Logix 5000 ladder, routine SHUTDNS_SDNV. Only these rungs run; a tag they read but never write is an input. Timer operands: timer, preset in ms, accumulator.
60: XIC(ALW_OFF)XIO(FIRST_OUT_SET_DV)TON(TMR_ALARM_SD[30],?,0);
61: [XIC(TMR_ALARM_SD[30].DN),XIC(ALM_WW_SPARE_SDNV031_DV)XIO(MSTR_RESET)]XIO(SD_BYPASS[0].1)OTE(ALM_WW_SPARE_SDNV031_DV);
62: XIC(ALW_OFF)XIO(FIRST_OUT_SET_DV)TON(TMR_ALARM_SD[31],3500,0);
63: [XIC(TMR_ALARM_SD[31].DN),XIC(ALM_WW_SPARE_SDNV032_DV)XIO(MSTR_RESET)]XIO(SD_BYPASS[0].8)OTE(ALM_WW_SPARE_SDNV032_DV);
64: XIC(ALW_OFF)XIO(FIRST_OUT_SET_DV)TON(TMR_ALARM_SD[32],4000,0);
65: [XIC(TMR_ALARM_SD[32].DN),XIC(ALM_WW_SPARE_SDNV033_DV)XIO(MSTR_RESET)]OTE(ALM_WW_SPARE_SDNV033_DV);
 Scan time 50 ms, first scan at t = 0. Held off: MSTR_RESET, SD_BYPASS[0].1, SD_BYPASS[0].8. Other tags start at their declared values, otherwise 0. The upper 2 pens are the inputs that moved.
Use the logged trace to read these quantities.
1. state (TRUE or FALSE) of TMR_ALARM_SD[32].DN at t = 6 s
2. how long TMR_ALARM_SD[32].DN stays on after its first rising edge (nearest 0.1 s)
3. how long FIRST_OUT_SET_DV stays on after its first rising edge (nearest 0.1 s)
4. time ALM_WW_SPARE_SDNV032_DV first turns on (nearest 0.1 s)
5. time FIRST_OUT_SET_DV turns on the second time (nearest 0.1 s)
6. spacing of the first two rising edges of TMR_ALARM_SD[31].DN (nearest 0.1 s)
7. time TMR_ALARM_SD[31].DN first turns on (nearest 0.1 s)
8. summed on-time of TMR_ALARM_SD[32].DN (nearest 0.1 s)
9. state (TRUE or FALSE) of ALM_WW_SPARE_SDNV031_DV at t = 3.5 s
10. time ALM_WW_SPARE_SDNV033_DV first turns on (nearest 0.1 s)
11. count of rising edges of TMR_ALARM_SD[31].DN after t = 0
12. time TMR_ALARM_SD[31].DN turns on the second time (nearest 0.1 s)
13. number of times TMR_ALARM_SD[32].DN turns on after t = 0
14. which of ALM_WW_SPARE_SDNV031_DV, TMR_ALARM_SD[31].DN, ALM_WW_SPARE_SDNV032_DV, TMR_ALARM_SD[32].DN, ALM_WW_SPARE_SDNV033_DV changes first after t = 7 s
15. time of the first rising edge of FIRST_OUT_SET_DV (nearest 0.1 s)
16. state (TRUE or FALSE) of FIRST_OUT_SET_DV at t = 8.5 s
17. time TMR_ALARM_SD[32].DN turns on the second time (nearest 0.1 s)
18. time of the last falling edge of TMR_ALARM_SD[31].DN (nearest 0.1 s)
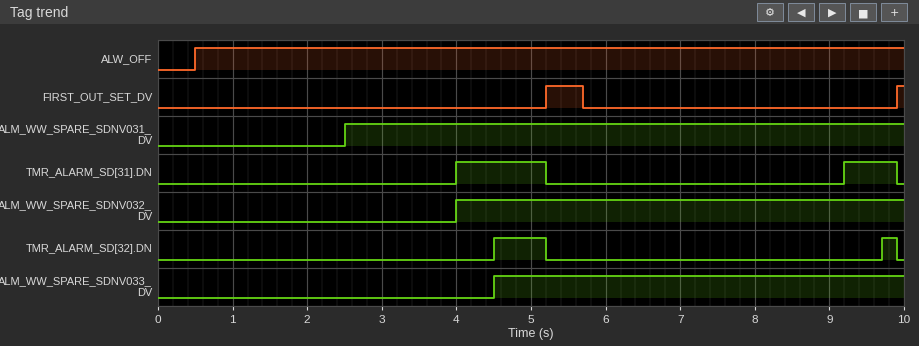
FALSE
0.7 s
0.5 s
4.0 s
9.9 s
5.2 s
4.0 s
0.9 s
TRUE
4.5 s
2
9.2 s
2
TMR_ALARM_SD[31].DN
5.2 s
FALSE
9.7 s
9.9 s
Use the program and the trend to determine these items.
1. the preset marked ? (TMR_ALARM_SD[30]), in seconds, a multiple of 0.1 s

2.0 s
